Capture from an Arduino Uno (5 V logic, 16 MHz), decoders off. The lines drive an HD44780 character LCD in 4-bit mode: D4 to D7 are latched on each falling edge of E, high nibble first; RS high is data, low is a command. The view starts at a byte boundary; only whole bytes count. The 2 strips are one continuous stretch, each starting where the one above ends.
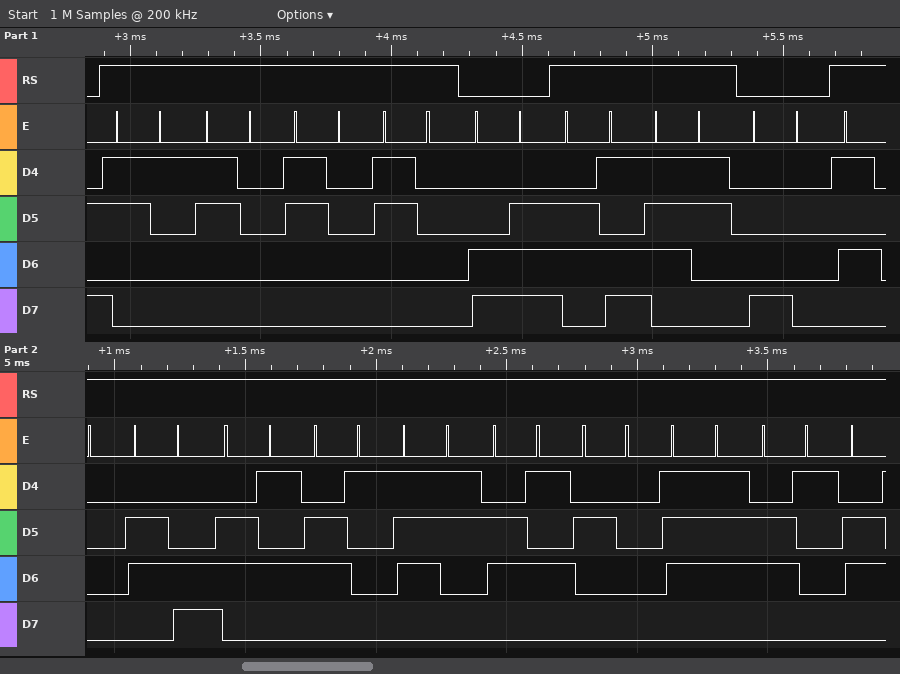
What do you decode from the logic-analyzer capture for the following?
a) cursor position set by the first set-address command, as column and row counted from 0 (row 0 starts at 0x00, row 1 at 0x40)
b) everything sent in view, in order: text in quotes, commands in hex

column 14, row 1
"1000" 0xCE "ms" 0x80 "Please wa"
